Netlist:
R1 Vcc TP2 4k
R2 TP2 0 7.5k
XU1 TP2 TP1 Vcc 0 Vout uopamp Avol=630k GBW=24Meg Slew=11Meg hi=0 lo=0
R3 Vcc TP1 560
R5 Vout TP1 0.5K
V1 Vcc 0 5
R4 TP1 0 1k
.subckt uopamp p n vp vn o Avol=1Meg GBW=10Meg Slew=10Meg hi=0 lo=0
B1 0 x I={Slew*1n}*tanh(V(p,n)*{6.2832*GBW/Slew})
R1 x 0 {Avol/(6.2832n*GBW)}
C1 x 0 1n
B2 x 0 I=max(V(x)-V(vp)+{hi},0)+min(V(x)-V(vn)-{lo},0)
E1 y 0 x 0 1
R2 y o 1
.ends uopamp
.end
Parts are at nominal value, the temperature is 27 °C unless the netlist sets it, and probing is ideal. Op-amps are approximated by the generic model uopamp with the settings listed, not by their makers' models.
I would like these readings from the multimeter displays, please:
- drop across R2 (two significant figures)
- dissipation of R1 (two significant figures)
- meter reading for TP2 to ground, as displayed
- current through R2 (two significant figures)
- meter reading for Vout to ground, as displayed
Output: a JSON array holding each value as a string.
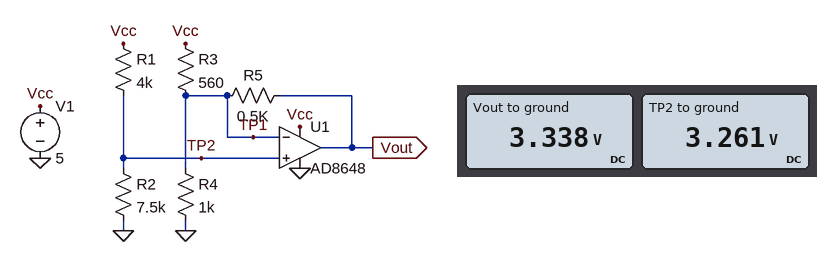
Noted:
["3.3 V", "760 µW", "3.261 V", "430 µA", "3.338 V"]
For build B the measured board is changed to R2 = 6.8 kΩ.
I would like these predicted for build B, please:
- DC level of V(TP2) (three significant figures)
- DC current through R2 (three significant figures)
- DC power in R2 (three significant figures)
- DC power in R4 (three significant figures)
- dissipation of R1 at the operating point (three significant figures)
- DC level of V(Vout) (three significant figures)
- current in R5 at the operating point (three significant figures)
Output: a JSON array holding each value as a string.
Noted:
["3.15 V", "463 µA", "1.46 mW", "9.91 mW", "857 µW", "3.07 V", "159 µA"]
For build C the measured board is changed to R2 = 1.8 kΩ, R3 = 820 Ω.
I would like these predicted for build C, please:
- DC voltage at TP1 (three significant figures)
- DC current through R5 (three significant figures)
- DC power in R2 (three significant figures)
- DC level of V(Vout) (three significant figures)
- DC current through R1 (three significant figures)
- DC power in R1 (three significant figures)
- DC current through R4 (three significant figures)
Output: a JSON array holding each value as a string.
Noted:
["1.55 V", "2.65 mA", "1.34 mW", "225 mV", "862 µA", "2.97 mW", "1.55 mA"]
